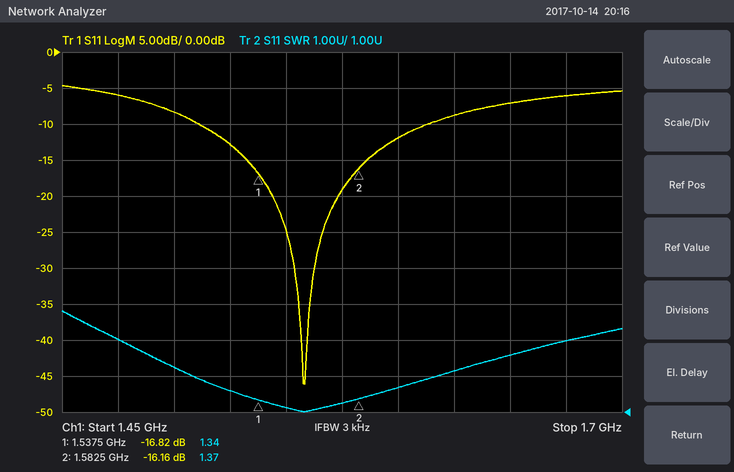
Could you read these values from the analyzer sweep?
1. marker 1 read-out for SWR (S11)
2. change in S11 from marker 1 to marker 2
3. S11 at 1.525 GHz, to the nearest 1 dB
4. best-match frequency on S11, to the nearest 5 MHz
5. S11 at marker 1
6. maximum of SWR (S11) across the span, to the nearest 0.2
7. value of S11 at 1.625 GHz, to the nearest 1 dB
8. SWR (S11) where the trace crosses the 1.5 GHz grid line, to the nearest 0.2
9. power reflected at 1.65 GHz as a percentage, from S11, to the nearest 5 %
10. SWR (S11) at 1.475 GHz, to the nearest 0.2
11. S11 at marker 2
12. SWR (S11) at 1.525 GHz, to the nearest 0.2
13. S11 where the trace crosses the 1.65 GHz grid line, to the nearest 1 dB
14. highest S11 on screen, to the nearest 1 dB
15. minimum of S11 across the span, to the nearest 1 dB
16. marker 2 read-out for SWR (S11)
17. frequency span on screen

1.34
0.66 dB
-13 dB
1.560 GHz
-16.82 dB
3.8
-9 dB
2.2
20 %
3.0
-16.16 dB
1.6
-7 dB
-5 dB
-46 dB
1.37
250 MHz
